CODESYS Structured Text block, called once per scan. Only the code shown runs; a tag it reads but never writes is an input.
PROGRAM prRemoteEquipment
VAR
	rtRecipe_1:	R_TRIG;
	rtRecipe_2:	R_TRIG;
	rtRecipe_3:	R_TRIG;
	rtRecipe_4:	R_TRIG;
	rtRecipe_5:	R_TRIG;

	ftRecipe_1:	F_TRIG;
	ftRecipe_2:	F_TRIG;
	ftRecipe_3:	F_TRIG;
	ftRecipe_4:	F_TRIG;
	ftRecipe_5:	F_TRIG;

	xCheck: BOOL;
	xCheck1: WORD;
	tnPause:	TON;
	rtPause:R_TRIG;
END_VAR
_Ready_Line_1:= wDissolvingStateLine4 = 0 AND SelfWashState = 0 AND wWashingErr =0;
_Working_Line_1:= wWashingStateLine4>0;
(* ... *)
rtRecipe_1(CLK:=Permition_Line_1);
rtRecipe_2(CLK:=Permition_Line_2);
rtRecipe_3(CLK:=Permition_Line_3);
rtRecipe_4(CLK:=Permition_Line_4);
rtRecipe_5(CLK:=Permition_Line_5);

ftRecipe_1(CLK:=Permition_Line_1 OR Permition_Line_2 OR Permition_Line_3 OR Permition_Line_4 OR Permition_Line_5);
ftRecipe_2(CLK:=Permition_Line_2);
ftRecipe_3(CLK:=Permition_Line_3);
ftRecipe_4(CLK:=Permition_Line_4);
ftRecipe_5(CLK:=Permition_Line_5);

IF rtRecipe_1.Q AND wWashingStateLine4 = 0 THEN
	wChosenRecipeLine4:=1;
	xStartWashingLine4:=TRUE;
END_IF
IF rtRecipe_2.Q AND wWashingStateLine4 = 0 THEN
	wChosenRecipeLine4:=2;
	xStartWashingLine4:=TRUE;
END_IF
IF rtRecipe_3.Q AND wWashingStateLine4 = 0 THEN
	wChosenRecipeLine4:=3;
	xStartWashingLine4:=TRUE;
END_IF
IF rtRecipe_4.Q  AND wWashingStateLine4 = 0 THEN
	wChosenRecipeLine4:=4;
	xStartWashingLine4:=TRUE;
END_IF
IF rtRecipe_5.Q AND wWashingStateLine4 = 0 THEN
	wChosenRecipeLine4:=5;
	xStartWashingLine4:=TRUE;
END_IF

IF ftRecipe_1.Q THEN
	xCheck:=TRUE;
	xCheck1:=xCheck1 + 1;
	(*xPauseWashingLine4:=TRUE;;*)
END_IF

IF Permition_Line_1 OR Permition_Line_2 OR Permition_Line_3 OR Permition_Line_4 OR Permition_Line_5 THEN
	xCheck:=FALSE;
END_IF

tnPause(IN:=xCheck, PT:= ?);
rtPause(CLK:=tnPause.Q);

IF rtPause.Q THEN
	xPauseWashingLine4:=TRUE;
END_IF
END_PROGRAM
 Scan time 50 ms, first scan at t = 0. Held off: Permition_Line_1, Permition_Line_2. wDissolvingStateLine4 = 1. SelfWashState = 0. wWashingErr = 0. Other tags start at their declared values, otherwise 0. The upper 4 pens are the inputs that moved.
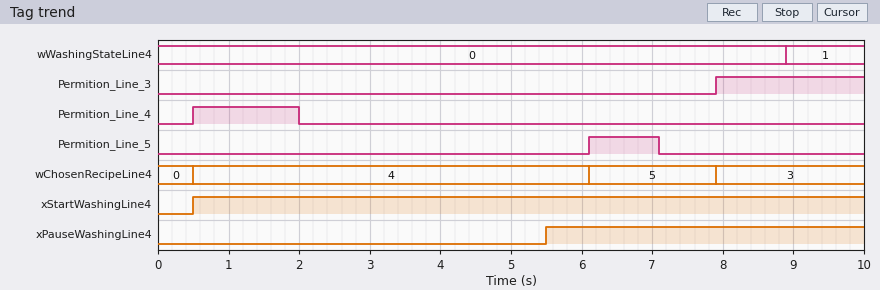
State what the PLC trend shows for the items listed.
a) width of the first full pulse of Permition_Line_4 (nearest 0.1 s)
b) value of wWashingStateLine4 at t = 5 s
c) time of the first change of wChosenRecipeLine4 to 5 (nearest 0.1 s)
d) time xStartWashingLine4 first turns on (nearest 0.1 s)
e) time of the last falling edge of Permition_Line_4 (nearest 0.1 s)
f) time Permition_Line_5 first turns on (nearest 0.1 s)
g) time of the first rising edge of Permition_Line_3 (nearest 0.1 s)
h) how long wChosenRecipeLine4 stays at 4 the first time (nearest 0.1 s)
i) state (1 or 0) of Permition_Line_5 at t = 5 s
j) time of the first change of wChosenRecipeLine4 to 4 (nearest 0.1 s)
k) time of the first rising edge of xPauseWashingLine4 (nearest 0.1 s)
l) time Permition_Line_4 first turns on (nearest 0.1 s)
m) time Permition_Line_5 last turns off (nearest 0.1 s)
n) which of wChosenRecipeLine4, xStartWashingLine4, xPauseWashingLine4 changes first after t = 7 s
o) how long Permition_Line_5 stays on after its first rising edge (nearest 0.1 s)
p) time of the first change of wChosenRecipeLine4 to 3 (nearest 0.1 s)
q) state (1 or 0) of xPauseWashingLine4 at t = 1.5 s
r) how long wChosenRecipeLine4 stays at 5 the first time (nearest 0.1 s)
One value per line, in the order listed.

1.5 s
0
6.1 s
0.5 s
2.0 s
6.1 s
7.9 s
5.6 s
0
0.5 s
5.5 s
0.5 s
7.1 s
wChosenRecipeLine4
1.0 s
7.9 s
0
1.8 s
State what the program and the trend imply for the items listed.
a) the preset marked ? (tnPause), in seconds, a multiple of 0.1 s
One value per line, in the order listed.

3.5 s
